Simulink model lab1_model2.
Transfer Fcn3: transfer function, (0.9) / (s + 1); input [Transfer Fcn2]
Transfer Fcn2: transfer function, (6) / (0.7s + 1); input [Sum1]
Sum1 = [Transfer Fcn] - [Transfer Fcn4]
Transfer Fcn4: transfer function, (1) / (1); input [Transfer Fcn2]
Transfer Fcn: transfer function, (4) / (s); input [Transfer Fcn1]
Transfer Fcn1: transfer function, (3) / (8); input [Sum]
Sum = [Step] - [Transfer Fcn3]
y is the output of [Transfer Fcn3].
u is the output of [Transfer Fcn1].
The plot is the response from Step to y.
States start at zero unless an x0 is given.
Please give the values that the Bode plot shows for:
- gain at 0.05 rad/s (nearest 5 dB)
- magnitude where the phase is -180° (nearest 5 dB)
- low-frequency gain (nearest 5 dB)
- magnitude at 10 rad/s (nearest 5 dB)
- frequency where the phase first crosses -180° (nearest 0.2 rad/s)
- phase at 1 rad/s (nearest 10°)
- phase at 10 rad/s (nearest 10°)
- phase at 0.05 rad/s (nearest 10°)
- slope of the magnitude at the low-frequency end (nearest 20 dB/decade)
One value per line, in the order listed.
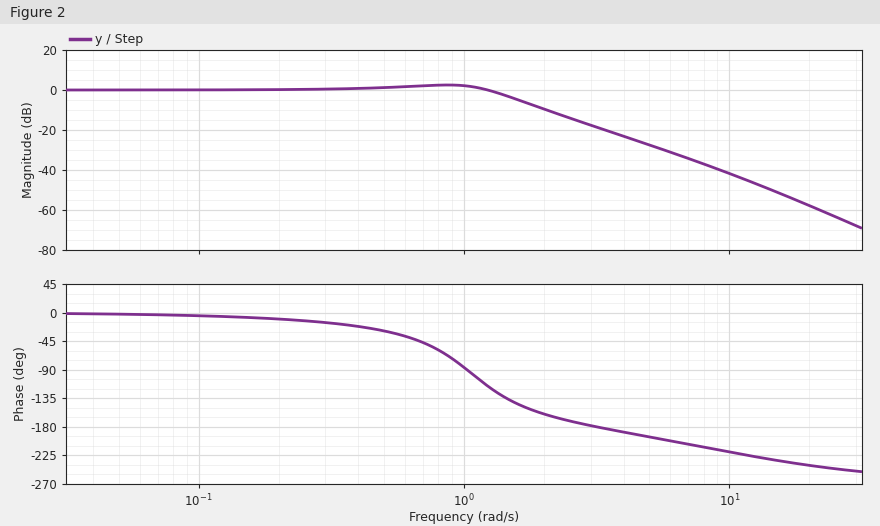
0 dB
-20 dB
0 dB
-40 dB
3.2 rad/s
-90°
-220°
0°
0 dB/decade
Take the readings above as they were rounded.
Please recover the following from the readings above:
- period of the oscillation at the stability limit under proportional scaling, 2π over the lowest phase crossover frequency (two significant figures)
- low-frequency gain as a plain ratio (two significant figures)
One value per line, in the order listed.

2.0 s
1.0
